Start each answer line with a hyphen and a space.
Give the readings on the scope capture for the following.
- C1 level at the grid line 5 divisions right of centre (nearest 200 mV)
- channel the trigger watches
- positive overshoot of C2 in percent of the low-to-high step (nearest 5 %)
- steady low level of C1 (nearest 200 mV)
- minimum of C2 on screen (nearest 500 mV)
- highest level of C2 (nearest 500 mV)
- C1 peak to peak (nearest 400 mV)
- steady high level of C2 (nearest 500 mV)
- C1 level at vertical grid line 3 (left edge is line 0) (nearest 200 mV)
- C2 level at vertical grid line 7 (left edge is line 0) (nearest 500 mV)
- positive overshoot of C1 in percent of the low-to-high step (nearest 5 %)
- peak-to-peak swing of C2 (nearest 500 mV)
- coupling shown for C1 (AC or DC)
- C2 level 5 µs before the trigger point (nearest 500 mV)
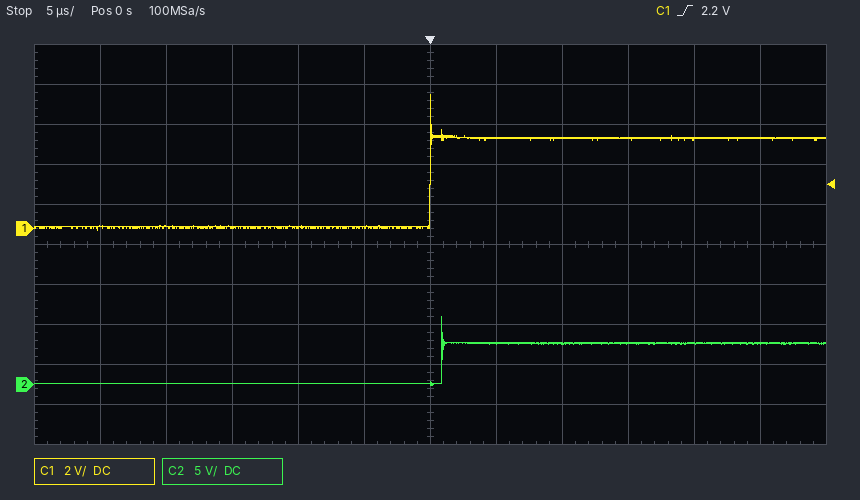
- 4.6 V
- C1
- 65 %
- 0.0 V
- 0.0 V
- 8.5 V
- 6.8 V
- 5.0 V
- 0.0 V
- 5.0 V
- 50 %
- 8.5 V
- DC
- 0.0 V
